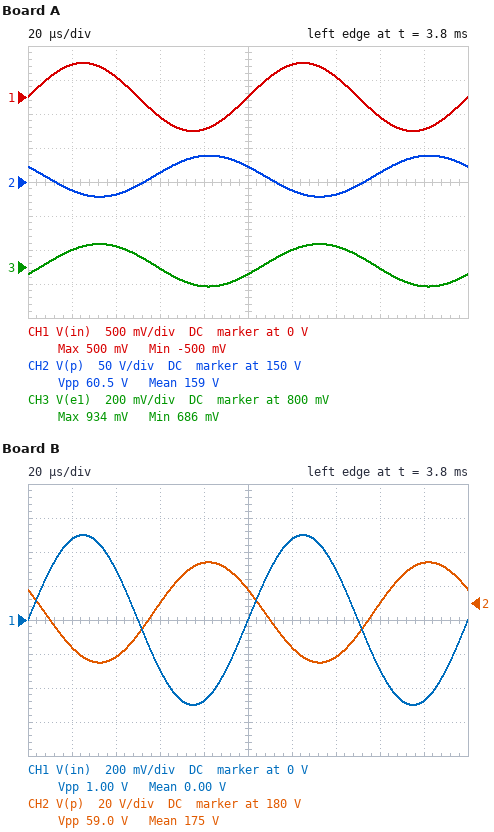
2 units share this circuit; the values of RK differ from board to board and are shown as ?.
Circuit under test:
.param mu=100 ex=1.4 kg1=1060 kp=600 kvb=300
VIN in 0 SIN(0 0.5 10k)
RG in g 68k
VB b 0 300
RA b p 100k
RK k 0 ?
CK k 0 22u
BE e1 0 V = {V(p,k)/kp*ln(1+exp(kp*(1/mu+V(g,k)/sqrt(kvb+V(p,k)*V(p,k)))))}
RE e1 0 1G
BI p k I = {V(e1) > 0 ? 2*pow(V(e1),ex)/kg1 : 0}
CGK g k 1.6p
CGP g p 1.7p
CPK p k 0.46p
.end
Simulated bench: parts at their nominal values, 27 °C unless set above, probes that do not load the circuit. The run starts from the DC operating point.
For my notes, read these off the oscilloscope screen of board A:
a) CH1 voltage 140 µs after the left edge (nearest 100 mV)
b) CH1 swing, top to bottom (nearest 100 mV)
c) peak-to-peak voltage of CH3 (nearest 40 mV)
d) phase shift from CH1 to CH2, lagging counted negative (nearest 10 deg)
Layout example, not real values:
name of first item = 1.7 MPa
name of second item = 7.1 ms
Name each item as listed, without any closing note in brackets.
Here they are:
CH1 voltage 140 µs after the left edge = 300 mV
CH1 swing, top to bottom = 1.0 V
peak-to-peak voltage of CH3 = 240 mV
phase shift from CH1 to CH2, lagging counted negative = 150 deg
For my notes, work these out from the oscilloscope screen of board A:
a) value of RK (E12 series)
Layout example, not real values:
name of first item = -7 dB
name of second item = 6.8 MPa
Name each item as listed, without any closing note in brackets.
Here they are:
value of RK = 560 Ω
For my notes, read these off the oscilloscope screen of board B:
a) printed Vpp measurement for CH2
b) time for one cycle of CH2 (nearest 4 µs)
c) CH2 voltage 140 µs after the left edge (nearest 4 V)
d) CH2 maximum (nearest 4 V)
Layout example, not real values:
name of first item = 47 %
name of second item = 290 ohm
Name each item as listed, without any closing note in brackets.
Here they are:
printed Vpp measurement for CH2 = 59.0 V
time for one cycle of CH2 = 100 µs
CH2 voltage 140 µs after the left edge = 148 V
CH2 maximum = 204 V
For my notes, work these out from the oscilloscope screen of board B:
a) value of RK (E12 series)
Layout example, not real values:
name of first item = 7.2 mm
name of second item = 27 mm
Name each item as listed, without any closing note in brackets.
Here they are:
value of RK = 820 Ω
